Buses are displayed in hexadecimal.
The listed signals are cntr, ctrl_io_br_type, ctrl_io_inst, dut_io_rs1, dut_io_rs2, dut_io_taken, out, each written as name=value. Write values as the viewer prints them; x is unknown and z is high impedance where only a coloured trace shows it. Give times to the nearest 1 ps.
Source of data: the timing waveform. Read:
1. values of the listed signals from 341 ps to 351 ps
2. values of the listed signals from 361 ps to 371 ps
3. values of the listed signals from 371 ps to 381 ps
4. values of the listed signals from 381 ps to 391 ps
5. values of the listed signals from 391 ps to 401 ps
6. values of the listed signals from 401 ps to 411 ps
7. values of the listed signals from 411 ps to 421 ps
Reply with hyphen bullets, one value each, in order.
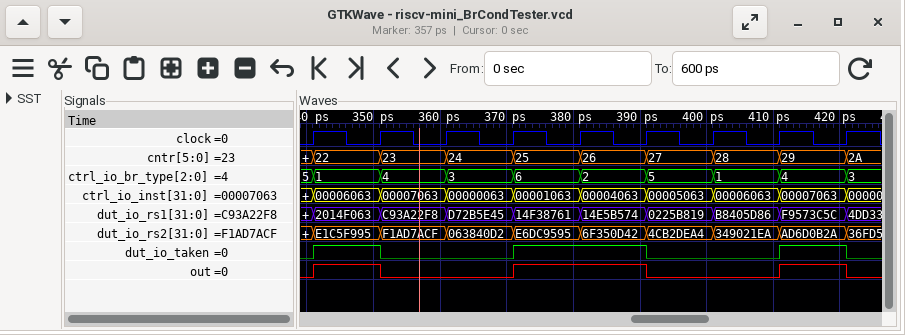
- cntr=22, ctrl_io_br_type=1, ctrl_io_inst=00006063, dut_io_rs1=2014F063, dut_io_rs2=E1C5F995, dut_io_taken=1, out=1
- cntr=24, ctrl_io_br_type=3, ctrl_io_inst=00000063, dut_io_rs1=D72B5E45, dut_io_rs2=063840D2, dut_io_taken=0, out=0
- cntr=25, ctrl_io_br_type=6, ctrl_io_inst=00001063, dut_io_rs1=14F38761, dut_io_rs2=E6DC9595, dut_io_taken=1, out=1
- cntr=26, ctrl_io_br_type=2, ctrl_io_inst=00004063, dut_io_rs1=14E5B574, dut_io_rs2=6F350D42, dut_io_taken=1, out=1
- cntr=27, ctrl_io_br_type=5, ctrl_io_inst=00005063, dut_io_rs1=0225B819, dut_io_rs2=4CB2DEA4, dut_io_taken=0, out=0
- cntr=28, ctrl_io_br_type=1, ctrl_io_inst=00006063, dut_io_rs1=B8405D86, dut_io_rs2=349021EA, dut_io_taken=0, out=0
- cntr=29, ctrl_io_br_type=4, ctrl_io_inst=00007063, dut_io_rs1=F9573C5C, dut_io_rs2=AD6D0B2A, dut_io_taken=1, out=1
